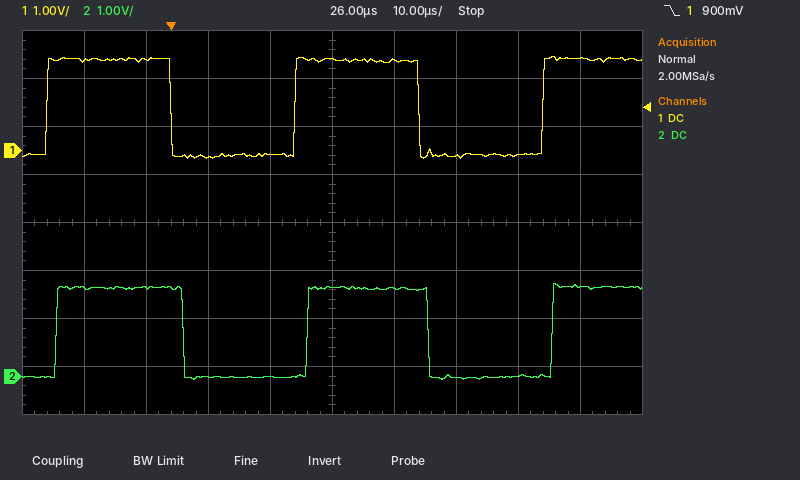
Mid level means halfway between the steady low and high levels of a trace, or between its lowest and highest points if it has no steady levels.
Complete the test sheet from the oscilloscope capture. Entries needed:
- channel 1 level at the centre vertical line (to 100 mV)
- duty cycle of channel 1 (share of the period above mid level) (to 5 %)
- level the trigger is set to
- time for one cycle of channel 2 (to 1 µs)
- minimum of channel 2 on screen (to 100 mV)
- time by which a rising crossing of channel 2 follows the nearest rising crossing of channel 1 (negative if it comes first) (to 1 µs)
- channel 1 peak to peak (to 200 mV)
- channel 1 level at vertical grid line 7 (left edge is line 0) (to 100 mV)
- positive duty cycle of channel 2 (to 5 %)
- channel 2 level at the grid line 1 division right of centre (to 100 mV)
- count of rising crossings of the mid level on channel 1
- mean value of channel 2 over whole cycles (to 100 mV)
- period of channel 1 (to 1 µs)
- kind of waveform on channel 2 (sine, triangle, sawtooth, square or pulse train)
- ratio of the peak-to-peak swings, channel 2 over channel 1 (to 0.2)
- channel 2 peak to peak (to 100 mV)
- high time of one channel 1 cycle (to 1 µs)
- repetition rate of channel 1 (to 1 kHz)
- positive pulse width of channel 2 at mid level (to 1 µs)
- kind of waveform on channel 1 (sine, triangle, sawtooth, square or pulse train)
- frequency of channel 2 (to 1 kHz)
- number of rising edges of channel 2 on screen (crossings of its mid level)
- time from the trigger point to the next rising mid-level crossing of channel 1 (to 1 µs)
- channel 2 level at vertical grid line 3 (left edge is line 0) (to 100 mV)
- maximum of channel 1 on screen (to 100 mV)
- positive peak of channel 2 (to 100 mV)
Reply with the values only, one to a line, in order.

1.9 V
50 %
900 mV
40 µs
-100 mV
+2 µs
2.2 V
-100 mV
50 %
1.8 V
3
900 mV
40 µs
square
1.0
2.0 V
20 µs
25 kHz
20 µs
square
25 kHz
3
20 µs
0.0 V
2.0 V
1.9 V
